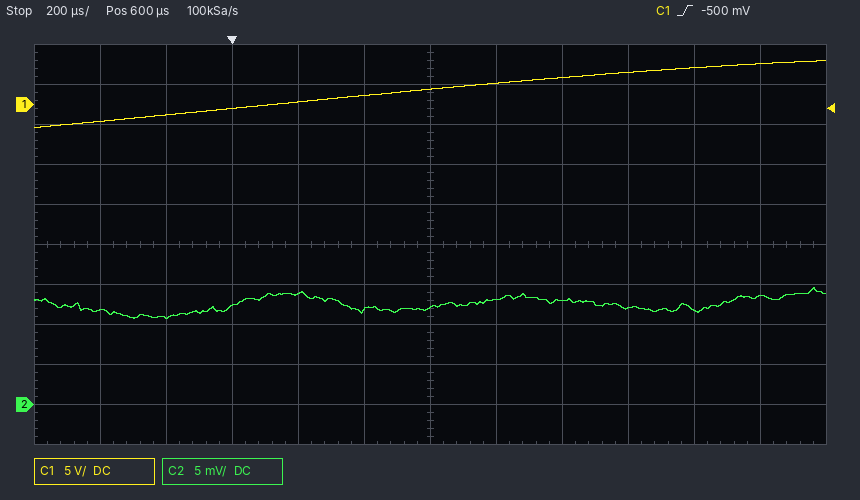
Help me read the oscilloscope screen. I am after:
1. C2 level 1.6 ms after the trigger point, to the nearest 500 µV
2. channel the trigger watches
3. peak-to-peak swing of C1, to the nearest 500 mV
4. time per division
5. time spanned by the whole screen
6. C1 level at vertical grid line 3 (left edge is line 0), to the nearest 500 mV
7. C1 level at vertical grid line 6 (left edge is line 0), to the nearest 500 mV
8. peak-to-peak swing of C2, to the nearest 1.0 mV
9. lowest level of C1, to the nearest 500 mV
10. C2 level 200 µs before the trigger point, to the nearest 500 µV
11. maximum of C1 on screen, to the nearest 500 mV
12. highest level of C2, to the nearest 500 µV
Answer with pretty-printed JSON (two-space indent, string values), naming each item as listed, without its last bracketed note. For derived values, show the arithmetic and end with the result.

{
  "C2 level 1.6 ms after the trigger point, to the nearest 500 µV": "13.5 mV",
  "channel the trigger watches": "C1",
  "peak-to-peak swing of C1, to the nearest 500 mV": "5.5 V − (-3.0 V) = 8.5 V",
  "time per division": "200 µs",
  "time spanned by the whole screen": "2.4 ms",
  "C1 level at vertical grid line 3 (left edge is line 0), to the nearest 500 mV": "-500 mV",
  "C1 level at vertical grid line 6 (left edge is line 0), to the nearest 500 mV": "2.0 V",
  "peak-to-peak swing of C2, to the nearest 1.0 mV": "4.0 mV",
  "lowest level of C1, to the nearest 500 mV": "-3.0 V",
  "C2 level 200 µs before the trigger point, to the nearest 500 µV": "11.0 mV",
  "maximum of C1 on screen, to the nearest 500 mV": "5.5 V",
  "highest level of C2, to the nearest 500 µV": "14.5 mV"
}
